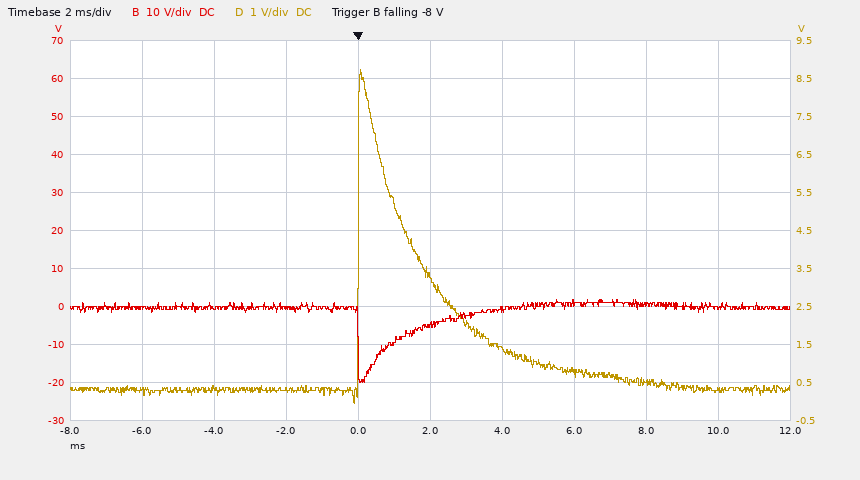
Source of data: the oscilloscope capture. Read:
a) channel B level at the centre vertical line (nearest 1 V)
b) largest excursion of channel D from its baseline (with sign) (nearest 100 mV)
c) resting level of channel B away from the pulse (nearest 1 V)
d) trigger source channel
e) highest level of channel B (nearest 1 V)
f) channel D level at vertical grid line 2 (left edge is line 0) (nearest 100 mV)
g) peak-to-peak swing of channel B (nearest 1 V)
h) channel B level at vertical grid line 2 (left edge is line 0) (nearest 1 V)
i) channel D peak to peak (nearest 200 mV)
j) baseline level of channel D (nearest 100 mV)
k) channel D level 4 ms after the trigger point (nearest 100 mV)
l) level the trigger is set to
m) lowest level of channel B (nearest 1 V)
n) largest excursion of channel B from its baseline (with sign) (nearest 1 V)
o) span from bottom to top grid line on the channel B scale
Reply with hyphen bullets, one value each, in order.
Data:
- -5 V
- +8.4 V
- 0 V
- channel B
- 2 V
- 300 mV
- 22 V
- 0 V
- 8.8 V
- 300 mV
- 1.4 V
- -8 V
- -20 V
- -20 V
- 100 V
